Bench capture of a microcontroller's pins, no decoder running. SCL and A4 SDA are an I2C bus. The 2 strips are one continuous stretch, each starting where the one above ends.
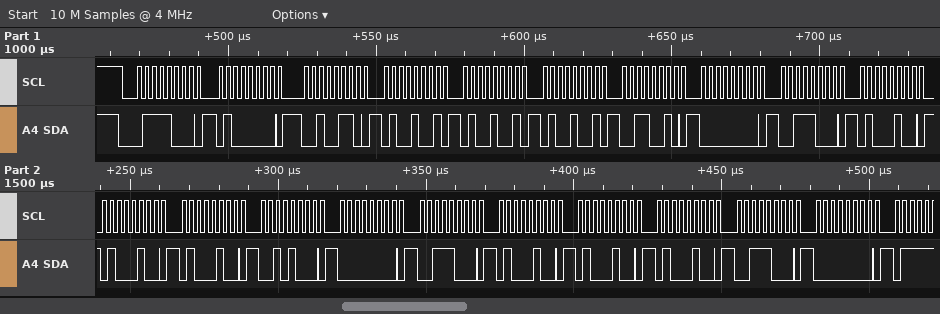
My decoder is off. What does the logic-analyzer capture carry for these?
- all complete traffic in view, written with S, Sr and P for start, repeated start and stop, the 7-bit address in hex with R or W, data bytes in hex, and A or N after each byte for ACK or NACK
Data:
S 3CW A 40 A 26 A 49 A 49 A 49 A 32 A 00 A 38 A 44 A 44 A 44 A 28 A 00 A 38 A 44 A 44 A 44 A 38 A 00 A
